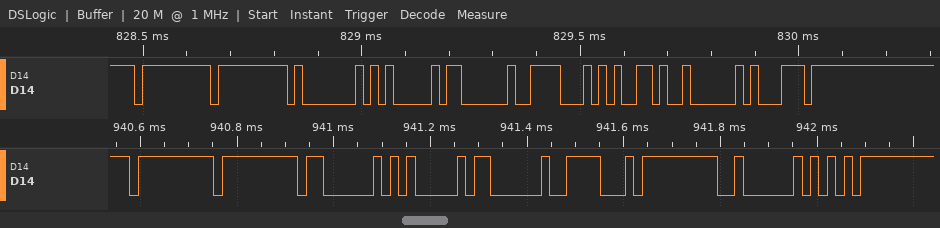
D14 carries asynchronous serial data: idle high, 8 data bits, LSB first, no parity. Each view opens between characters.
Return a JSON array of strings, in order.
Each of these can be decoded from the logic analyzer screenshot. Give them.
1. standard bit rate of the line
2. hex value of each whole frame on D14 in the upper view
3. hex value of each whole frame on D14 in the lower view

["57600 baud", "FF, FF, 01, 05, 03, 1E, 65, 02, 71", "FF, FF, 03, 05, 03, 1E, FF, 02, D5"]
